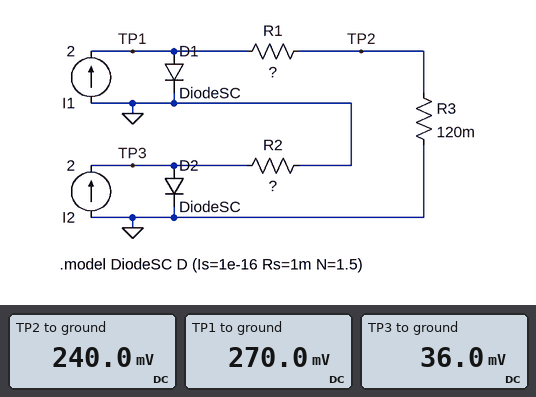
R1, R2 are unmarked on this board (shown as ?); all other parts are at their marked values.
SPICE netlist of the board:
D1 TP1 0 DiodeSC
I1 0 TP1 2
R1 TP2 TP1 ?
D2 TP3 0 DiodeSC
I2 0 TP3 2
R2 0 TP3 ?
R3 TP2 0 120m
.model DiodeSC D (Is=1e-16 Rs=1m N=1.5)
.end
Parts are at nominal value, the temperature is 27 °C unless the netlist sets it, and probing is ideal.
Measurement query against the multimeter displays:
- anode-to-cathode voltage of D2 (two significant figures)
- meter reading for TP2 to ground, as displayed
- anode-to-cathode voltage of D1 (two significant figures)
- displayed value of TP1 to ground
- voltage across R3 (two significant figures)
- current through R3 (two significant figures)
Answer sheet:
36 mV
240.0 mV
270 mV
270.0 mV
240 mV
2.0 A
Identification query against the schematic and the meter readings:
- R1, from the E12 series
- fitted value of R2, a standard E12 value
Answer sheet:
0.015 Ω
0.018 Ω
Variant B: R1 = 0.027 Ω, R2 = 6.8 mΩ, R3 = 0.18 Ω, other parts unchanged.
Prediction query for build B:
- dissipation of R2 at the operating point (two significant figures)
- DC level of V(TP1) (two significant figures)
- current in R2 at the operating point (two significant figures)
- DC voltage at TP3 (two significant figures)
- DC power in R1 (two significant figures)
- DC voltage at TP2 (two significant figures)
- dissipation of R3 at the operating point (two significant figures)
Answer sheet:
27 mW
410 mV
2.0 A
14 mV
110 mW
360 mV
720 mW
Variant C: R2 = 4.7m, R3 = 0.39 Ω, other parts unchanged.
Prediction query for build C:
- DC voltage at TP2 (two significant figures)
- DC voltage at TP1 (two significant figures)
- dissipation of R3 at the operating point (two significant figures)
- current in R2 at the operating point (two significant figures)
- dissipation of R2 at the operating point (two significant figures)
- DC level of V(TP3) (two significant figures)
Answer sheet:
780 mV
810 mV
1.6 W
2.0 A
19 mW
9.4 mV
